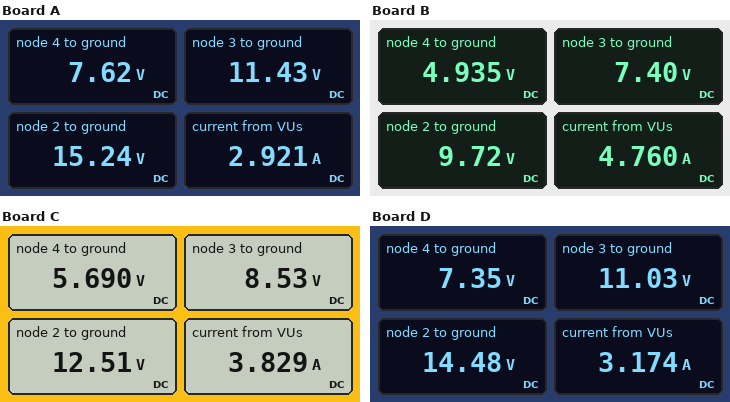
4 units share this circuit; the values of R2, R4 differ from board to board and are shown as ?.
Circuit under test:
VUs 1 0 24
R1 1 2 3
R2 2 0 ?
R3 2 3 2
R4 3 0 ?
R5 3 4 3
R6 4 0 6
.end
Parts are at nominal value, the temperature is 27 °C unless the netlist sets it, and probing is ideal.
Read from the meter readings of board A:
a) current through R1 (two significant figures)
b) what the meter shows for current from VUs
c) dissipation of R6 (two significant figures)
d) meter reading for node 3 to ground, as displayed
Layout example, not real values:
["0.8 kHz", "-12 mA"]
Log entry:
["2.9 A", "2.921 A", "9.7 W", "11.43 V"]
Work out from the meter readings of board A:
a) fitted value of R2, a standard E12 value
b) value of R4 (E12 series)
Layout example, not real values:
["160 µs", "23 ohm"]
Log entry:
["15 Ω", "18 Ω"]
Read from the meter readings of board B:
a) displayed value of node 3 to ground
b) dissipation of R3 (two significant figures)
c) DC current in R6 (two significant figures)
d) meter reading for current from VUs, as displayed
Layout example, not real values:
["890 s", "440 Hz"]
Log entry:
["7.40 V", "2.7 W", "820 mA", "4.760 A"]
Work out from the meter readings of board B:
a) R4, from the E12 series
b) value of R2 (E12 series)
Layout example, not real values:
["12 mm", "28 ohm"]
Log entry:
["22 Ω", "2.7 Ω"]
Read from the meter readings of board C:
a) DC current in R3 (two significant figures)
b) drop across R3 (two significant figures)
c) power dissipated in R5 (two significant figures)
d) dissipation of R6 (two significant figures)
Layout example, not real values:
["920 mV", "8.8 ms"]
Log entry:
["2.0 A", "4.0 V", "2.7 W", "5.4 W"]
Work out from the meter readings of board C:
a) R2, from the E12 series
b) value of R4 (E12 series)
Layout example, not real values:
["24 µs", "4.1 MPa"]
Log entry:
["6.8 Ω", "8.2 Ω"]
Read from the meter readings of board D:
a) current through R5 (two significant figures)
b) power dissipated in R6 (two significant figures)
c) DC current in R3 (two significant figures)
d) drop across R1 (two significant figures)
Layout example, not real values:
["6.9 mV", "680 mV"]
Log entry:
["1.2 A", "9.0 W", "1.7 A", "9.5 V"]
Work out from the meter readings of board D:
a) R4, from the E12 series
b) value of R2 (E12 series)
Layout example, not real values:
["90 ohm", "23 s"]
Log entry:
["22 Ω", "10 Ω"]
